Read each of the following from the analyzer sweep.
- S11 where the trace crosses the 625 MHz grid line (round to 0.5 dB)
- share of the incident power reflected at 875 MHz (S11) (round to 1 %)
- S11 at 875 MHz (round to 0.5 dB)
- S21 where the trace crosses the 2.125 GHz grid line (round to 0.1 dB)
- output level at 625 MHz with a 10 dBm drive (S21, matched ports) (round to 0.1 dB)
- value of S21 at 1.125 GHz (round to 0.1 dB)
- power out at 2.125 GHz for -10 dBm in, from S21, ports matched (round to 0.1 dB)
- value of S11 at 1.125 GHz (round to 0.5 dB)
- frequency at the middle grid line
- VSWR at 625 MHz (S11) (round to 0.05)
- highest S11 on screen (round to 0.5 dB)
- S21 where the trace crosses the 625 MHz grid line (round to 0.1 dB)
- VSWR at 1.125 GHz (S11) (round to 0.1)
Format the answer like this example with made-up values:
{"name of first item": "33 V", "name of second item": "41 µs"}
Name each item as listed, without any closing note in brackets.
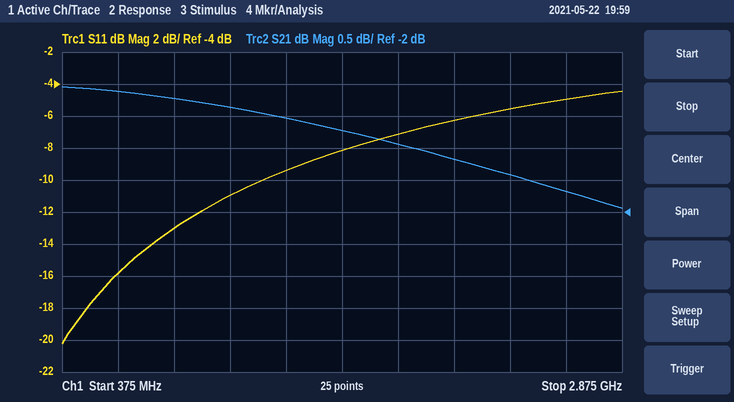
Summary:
{"S11 where the trace crosses the 625 MHz grid line": "-16.0 dB", "share of the incident power reflected at 875 MHz (S11)": "5 %", "S11 at 875 MHz": "-13.0 dB", "S21 where the trace crosses the 2.125 GHz grid line": "-1.2 dB", "output level at 625 MHz with a 10 dBm drive (S21, matched ports)": "9.9 dBm", "value of S21 at 1.125 GHz": "-0.4 dB", "power out at 2.125 GHz for -10 dBm in, from S21, ports matched": "-11.2 dBm", "value of S11 at 1.125 GHz": "-11.0 dB", "frequency at the middle grid line": "1.625 GHz", "VSWR at 625 MHz (S11)": "1.40", "highest S11 on screen": "-4.5 dB", "S21 where the trace crosses the 625 MHz grid line": "-0.1 dB", "VSWR at 1.125 GHz (S11)": "1.8"}
